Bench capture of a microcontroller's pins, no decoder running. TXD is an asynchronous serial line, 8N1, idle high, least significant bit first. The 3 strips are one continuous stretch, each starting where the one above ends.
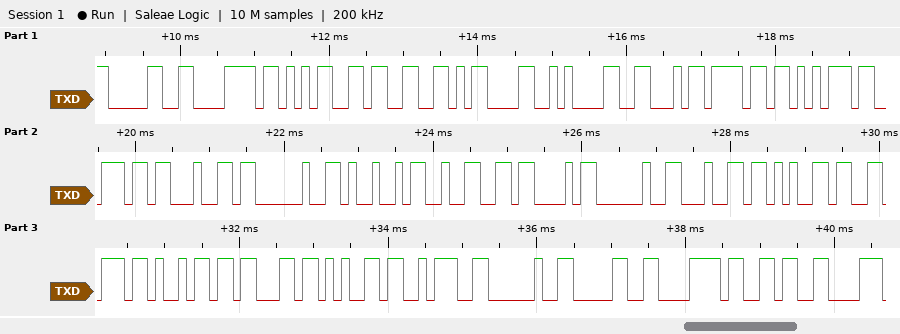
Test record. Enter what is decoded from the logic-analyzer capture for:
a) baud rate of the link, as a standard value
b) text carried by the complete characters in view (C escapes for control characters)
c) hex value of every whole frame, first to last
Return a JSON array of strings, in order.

["9600 baud", "\"0x53\\r\\nFound I2C device: 0x6\"", "30 78 35 33 0D 0A 46 6F 75 6E 64 20 49 32 43 20 64 65 76 69 63 65 3A 20 30 78 36"]
